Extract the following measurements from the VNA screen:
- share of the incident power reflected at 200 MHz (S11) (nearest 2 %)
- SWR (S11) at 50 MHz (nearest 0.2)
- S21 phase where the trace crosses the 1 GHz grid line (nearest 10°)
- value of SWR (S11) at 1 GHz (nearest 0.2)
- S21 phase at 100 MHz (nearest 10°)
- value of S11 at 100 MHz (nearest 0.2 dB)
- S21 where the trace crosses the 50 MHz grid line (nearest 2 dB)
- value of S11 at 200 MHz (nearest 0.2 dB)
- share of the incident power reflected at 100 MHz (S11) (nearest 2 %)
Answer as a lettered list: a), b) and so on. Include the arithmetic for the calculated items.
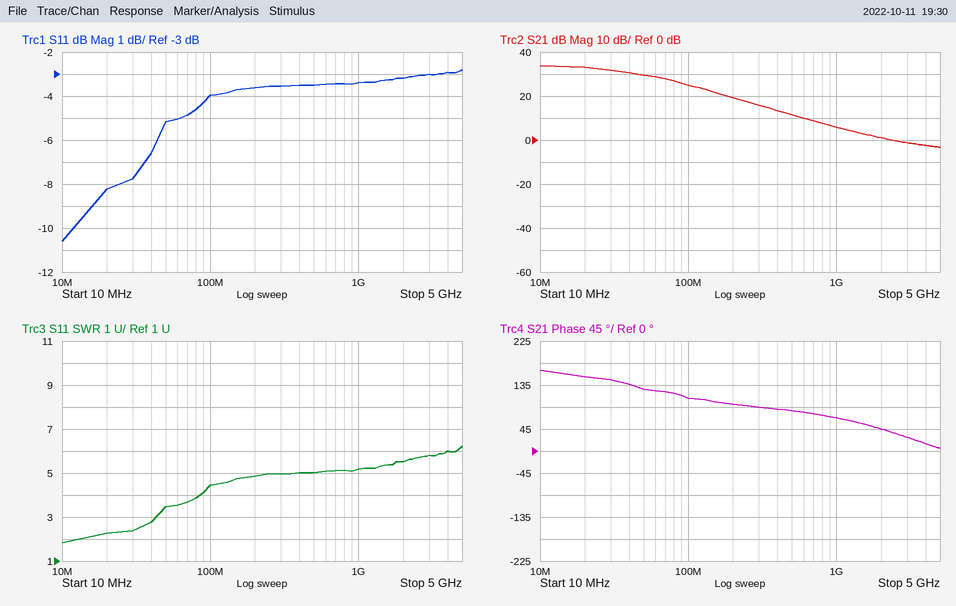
a) 10^(-3.6/10) ≈ 44 %
b) 3.4
c) 70°
d) 5.2
e) 110°
f) -4.0 dB
g) 30 dB
h) -3.6 dB
i) 10^(-4/10) ≈ 40 %
